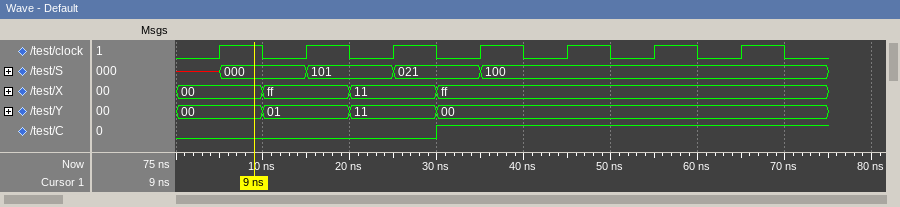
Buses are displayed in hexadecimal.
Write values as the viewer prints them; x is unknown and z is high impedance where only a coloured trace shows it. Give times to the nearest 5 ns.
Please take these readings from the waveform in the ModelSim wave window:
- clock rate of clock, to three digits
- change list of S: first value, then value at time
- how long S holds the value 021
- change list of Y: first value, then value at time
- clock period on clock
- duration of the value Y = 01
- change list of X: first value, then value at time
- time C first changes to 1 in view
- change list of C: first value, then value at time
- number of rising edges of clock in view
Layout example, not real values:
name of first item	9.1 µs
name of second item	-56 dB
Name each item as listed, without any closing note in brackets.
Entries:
clock rate of clock, to three digits	100 MHz
change list of S: first value, then value at time	x, 000 at 5 ns, 101 at 15 ns, 021 at 25 ns, 100 at 35 ns
how long S holds the value 021	10 ns
change list of Y: first value, then value at time	00, 01 at 10 ns, 11 at 20 ns, 00 at 30 ns
clock period on clock	10 ns
duration of the value Y = 01	10 ns
change list of X: first value, then value at time	00, ff at 10 ns, 11 at 20 ns, ff at 30 ns
time C first changes to 1 in view	30 ns
change list of C: first value, then value at time	0, 1 at 30 ns
number of rising edges of clock in view	7
